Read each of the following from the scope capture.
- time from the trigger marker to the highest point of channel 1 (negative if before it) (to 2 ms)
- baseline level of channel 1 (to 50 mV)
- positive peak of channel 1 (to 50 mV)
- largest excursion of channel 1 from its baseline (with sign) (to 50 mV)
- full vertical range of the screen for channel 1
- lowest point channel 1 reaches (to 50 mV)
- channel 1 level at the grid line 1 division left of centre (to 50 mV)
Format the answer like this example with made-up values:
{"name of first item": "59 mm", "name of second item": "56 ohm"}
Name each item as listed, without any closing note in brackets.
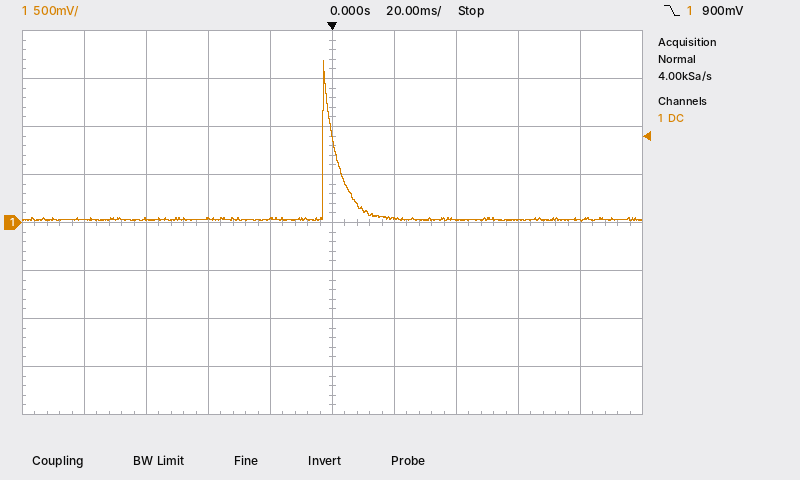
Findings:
{"time from the trigger marker to the highest point of channel 1 (negative if before it)": "-2 ms", "baseline level of channel 1": "50 mV", "positive peak of channel 1": "1.70 V", "largest excursion of channel 1 from its baseline (with sign)": "+1.65 V", "full vertical range of the screen for channel 1": "4 V", "lowest point channel 1 reaches": "0 mV", "channel 1 level at the grid line 1 division left of centre": "50 mV"}
